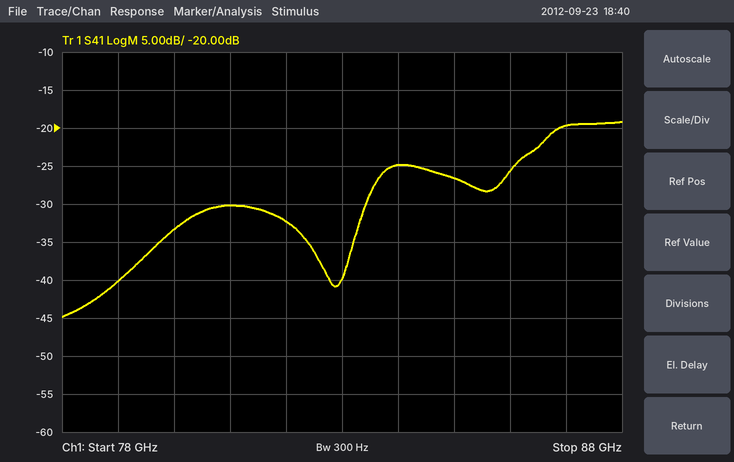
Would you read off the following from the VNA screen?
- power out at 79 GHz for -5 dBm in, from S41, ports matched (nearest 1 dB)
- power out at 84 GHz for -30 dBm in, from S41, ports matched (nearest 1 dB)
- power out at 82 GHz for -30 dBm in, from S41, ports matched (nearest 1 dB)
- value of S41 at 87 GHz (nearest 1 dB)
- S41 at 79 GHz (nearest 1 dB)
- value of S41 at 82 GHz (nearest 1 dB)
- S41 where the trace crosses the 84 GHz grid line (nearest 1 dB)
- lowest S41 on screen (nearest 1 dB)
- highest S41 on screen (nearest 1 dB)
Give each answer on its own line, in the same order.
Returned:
-45 dBm
-55 dBm
-62 dBm
-20 dB
-40 dB
-32 dB
-25 dB
-45 dB
-19 dB
